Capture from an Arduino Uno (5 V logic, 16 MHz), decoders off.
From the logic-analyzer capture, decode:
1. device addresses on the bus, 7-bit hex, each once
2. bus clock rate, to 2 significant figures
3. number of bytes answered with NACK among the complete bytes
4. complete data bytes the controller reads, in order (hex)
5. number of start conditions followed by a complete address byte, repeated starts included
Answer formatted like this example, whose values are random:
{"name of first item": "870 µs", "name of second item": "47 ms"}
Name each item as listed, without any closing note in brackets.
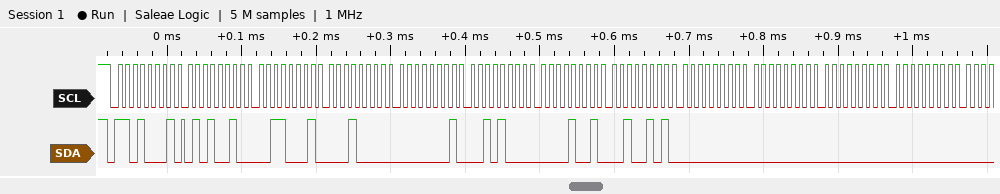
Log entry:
{"device addresses on the bus, 7-bit hex, each once": "0x68", "bus clock rate, to 2 significant figures": "100 kHz", "number of bytes answered with NACK among the complete bytes": "0", "complete data bytes the controller reads, in order": "52 31 10 01 28 09 25 00 00 00 00", "number of start conditions followed by a complete address byte, repeated starts included": "1"}
